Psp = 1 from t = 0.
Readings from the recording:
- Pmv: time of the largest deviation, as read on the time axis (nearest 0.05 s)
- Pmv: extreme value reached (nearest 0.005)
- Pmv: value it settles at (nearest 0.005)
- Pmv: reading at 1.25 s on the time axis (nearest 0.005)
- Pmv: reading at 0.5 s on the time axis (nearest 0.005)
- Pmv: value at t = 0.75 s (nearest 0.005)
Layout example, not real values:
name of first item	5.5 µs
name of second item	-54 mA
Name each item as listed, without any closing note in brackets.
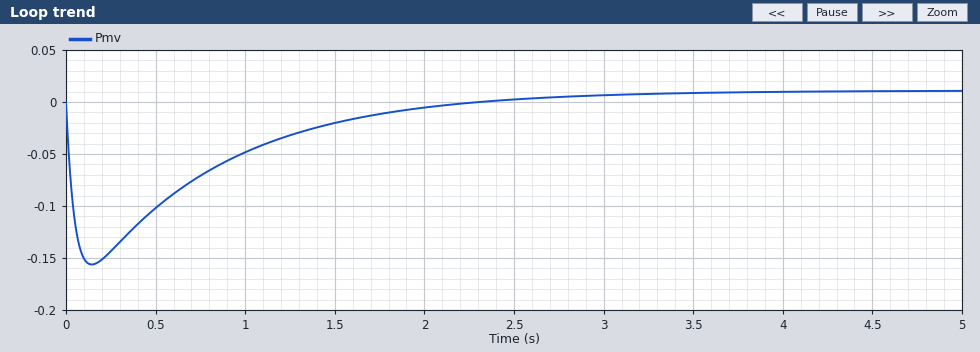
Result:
Pmv: time of the largest deviation, as read on the time axis	0.15 s
Pmv: extreme value reached	-0.155
Pmv: value it settles at	0.010
Pmv: reading at 1.25 s on the time axis	-0.030
Pmv: reading at 0.5 s on the time axis	-0.100
Pmv: value at t = 0.75 s	-0.070
